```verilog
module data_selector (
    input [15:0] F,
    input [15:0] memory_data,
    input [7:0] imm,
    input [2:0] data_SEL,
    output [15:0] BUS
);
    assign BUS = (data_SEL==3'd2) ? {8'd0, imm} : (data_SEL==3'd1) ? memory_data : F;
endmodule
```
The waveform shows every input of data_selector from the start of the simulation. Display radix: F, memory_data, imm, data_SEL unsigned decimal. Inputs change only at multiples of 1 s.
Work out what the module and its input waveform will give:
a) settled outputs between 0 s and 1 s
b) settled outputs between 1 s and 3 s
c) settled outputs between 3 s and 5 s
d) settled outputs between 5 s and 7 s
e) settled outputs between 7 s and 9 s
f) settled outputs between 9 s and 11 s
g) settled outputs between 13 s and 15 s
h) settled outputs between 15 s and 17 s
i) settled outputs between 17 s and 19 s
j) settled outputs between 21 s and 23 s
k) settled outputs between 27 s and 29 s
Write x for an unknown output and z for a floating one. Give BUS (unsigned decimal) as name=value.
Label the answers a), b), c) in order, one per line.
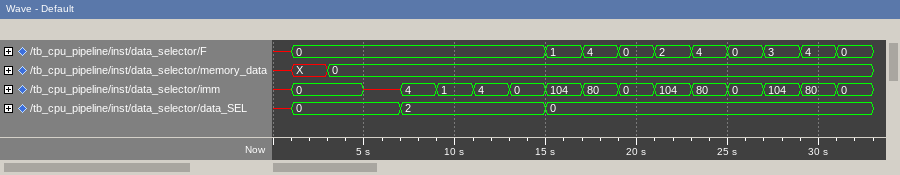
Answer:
a) BUS=x
b) BUS=0
c) BUS=0
d) BUS=0
e) BUS=4
f) BUS=1
g) BUS=0
h) BUS=1
i) BUS=4
j) BUS=2
k) BUS=3
